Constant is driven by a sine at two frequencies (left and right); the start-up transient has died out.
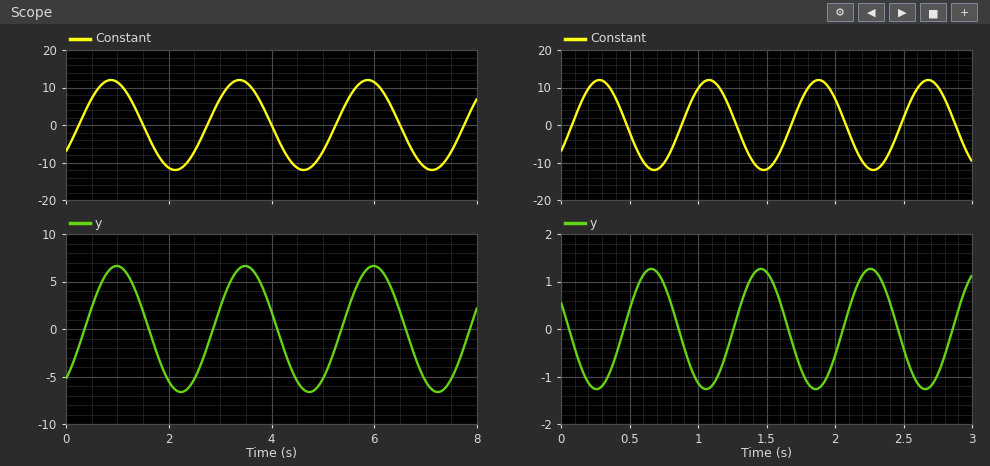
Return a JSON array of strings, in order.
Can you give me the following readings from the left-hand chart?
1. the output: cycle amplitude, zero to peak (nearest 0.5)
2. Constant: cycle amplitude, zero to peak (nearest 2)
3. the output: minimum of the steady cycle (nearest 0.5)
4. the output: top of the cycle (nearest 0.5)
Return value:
["6.5", "12", "-6.5", "6.5"]
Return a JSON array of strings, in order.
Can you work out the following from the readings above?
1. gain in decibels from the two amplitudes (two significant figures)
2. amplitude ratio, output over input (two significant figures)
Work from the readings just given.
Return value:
["-5.3 dB", "0.54"]
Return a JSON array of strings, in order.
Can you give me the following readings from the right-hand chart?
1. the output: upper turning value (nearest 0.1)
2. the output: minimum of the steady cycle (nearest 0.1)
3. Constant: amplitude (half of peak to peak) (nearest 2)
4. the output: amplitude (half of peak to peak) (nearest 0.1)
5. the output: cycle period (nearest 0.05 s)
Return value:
["1.3", "-1.3", "12", "1.3", "0.80 s"]
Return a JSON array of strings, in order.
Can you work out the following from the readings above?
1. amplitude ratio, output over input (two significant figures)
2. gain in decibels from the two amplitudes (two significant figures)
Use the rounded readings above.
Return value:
["0.11", "-19 dB"]
